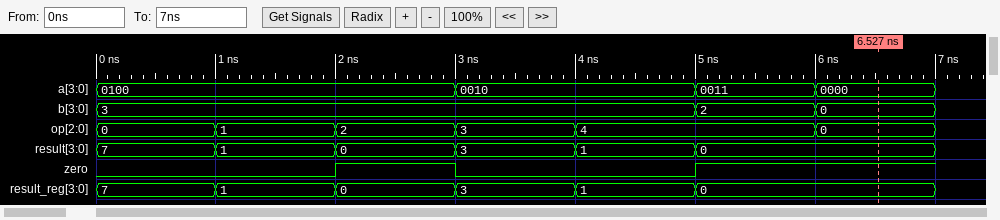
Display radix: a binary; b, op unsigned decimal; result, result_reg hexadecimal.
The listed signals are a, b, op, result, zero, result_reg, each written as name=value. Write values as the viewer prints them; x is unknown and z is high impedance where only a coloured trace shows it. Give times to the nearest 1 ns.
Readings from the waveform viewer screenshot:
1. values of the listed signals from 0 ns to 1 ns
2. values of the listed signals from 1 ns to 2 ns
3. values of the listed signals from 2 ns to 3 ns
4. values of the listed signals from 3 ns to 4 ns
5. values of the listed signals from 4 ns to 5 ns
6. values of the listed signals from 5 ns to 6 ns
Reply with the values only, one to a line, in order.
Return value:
a=0100, b=3, op=0, result=7, zero=0, result_reg=7
a=0100, b=3, op=1, result=1, zero=0, result_reg=1
a=0100, b=3, op=2, result=0, zero=1, result_reg=0
a=0010, b=3, op=3, result=3, zero=0, result_reg=3
a=0010, b=3, op=4, result=1, zero=0, result_reg=1
a=0011, b=2, op=4, result=0, zero=1, result_reg=0
